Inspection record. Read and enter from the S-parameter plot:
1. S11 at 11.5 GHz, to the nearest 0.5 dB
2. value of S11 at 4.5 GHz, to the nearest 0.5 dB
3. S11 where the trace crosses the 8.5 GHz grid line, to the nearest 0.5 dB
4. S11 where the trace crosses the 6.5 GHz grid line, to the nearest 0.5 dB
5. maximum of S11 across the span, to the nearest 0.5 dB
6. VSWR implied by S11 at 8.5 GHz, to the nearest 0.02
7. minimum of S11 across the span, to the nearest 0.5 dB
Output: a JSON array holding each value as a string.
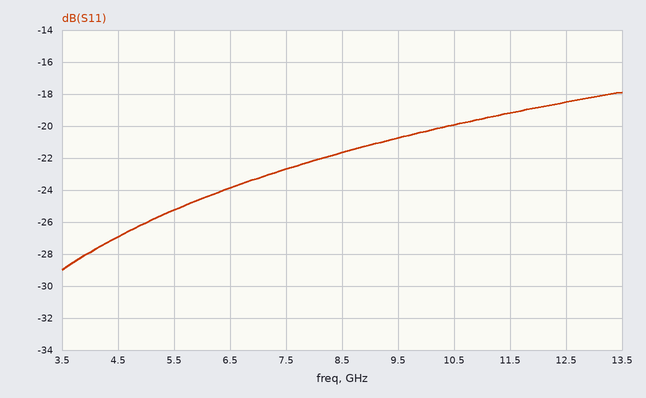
["-19.0 dB", "-27.0 dB", "-21.5 dB", "-24.0 dB", "-18.0 dB", "1.18", "-29.0 dB"]
